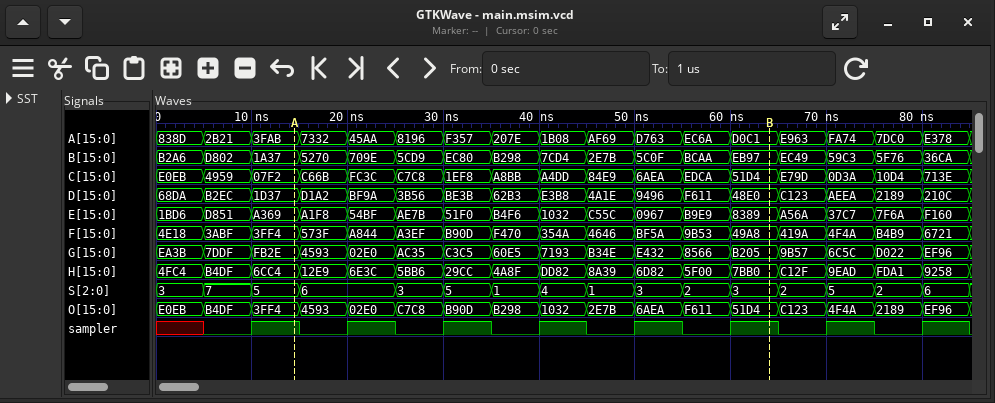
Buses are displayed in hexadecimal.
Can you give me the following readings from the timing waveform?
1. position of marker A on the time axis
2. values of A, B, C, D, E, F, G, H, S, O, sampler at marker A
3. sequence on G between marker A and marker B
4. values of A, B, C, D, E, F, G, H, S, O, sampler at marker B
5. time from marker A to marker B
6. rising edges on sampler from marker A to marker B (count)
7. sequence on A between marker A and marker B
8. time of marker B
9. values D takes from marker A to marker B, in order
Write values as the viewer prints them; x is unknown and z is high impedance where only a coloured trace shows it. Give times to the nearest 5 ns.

15 ns
A=3FAB, B=1A37, C=07F2, D=1D37, E=A369, F=3FF4, G=FB2E, H=6CC4, S=5, O=3FF4, sampler=1
FB2E, 4593, 02E0, AC35, C3C5, 60E5, 7193, B34E, E432, 8566, B205
A=D0C1, B=EB97, C=51D4, D=48E0, E=8389, F=49A8, G=B205, H=7BB0, S=3, O=51D4, sampler=1
50 ns
5
3FAB, 7332, 45AA, 8196, F357, 207E, 1B08, AF69, D763, EC6A, D0C1
65 ns
1D37, D1A2, BF9A, 3B56, BE3B, 62B3, E3B8, 4A1E, 9496, F611, 48E0
